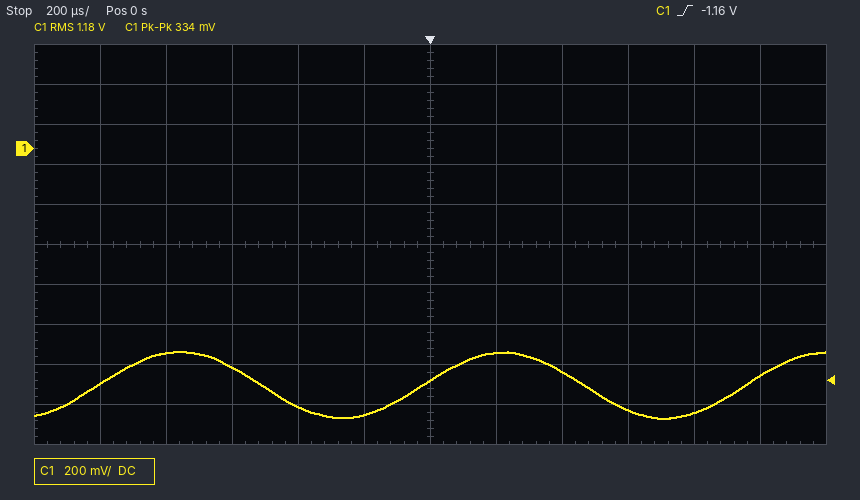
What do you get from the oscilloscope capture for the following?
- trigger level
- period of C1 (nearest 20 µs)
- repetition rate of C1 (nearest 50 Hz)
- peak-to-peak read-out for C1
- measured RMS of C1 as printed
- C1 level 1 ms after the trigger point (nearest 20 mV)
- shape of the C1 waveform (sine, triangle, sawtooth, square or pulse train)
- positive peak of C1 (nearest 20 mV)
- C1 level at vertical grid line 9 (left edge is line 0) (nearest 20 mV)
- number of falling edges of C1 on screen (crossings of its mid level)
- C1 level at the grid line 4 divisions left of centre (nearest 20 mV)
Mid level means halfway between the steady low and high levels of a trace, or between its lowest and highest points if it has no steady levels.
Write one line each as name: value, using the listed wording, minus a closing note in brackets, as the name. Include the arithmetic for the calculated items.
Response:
trigger level: -1.16 V
period of C1: 980 µs
repetition rate of C1: 1 / 980 µs ≈ 1.02 kHz, so 1.00 kHz to the nearest 50 Hz
peak-to-peak read-out for C1: 334 mV
measured RMS of C1 as printed: 1.18 V
C1 level 1 ms after the trigger point: -1.14 V
shape of the C1 waveform: sine
positive peak of C1: -1.02 V
C1 level at vertical grid line 9 (left edge is line 0): -1.30 V
number of falling edges of C1 on screen: 2
C1 level at the grid line 4 divisions left of centre: -1.02 V
